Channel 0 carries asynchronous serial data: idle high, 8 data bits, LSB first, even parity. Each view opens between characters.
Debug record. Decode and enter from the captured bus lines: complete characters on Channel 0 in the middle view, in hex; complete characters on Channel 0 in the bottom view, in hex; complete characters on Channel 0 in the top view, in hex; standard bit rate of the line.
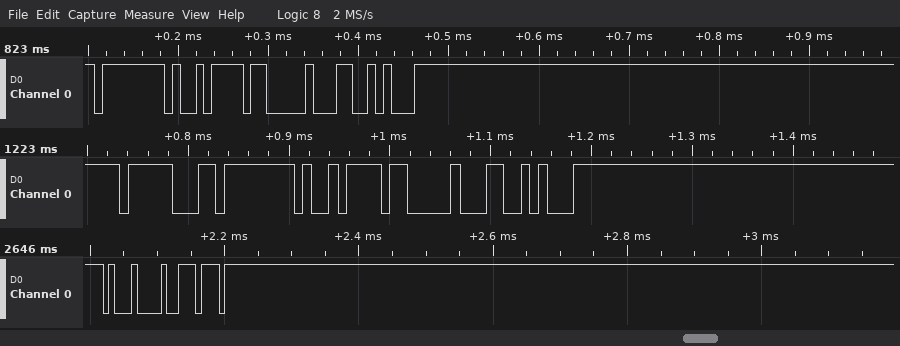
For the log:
1F, FF, 7A, 10, 8A
11, EE
FF, 7A, 10, 8A
115200 baud
